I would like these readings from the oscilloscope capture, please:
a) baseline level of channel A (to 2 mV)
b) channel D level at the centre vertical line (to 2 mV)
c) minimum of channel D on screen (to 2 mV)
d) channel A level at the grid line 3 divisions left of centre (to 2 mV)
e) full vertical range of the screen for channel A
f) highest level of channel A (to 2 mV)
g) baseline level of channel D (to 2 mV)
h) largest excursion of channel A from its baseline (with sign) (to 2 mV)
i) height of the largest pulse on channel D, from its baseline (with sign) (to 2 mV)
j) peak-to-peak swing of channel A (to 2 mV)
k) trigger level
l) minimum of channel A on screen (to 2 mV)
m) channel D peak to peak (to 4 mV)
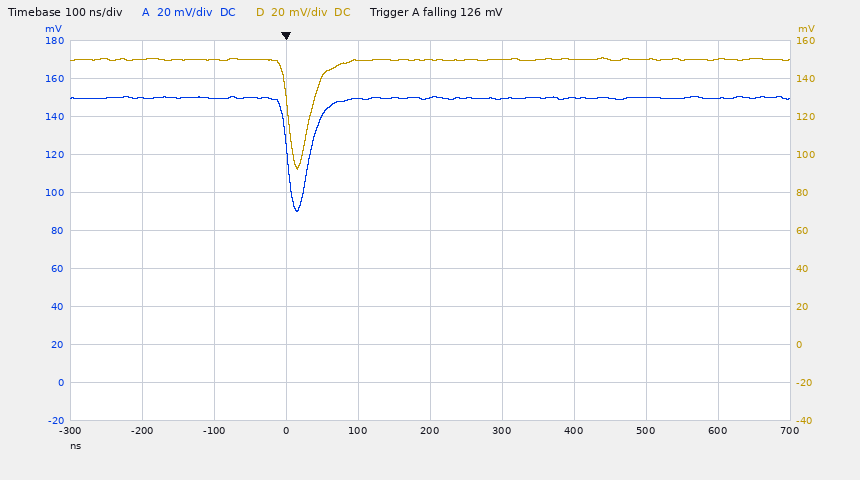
150 mV
150 mV
92 mV
150 mV
200 mV
150 mV
150 mV
-60 mV
-58 mV
60 mV
126 mV
90 mV
60 mV
